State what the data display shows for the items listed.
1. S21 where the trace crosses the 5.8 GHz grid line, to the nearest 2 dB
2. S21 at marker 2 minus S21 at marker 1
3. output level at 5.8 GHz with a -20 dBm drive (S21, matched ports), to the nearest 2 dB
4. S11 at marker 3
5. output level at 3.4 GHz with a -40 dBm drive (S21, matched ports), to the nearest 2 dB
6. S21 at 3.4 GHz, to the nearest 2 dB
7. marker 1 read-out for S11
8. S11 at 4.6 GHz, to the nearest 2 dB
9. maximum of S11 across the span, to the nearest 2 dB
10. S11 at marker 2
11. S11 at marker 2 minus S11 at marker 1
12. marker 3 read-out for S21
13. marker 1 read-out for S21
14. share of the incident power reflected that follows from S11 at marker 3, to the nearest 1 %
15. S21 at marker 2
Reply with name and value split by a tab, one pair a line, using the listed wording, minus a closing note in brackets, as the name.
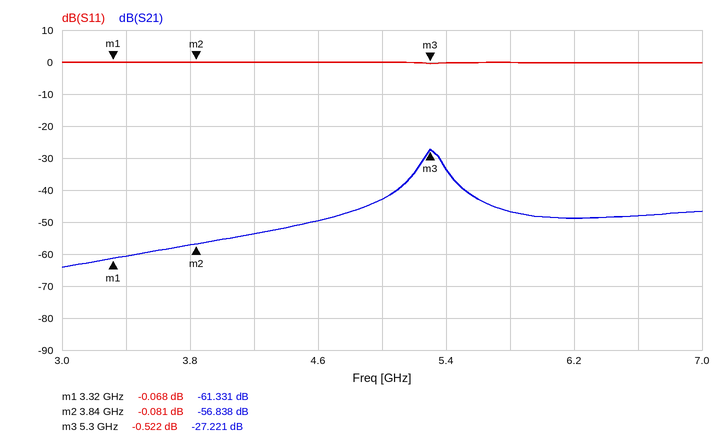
S21 where the trace crosses the 5.8 GHz grid line, to the nearest 2 dB	-46 dB
S21 at marker 2 minus S21 at marker 1	4.493 dB
output level at 5.8 GHz with a -20 dBm drive (S21, matched ports), to the nearest 2 dB	-66 dBm
S11 at marker 3	-0.522 dB
output level at 3.4 GHz with a -40 dBm drive (S21, matched ports), to the nearest 2 dB	-100 dBm
S21 at 3.4 GHz, to the nearest 2 dB	-60 dB
marker 1 read-out for S11	-0.068 dB
S11 at 4.6 GHz, to the nearest 2 dB	0 dB
maximum of S11 across the span, to the nearest 2 dB	0 dB
S11 at marker 2	-0.081 dB
S11 at marker 2 minus S11 at marker 1	-0.013 dB
marker 3 read-out for S21	-27.221 dB
marker 1 read-out for S21	-61.331 dB
share of the incident power reflected that follows from S11 at marker 3, to the nearest 1 %	89 %
S21 at marker 2	-56.838 dB
